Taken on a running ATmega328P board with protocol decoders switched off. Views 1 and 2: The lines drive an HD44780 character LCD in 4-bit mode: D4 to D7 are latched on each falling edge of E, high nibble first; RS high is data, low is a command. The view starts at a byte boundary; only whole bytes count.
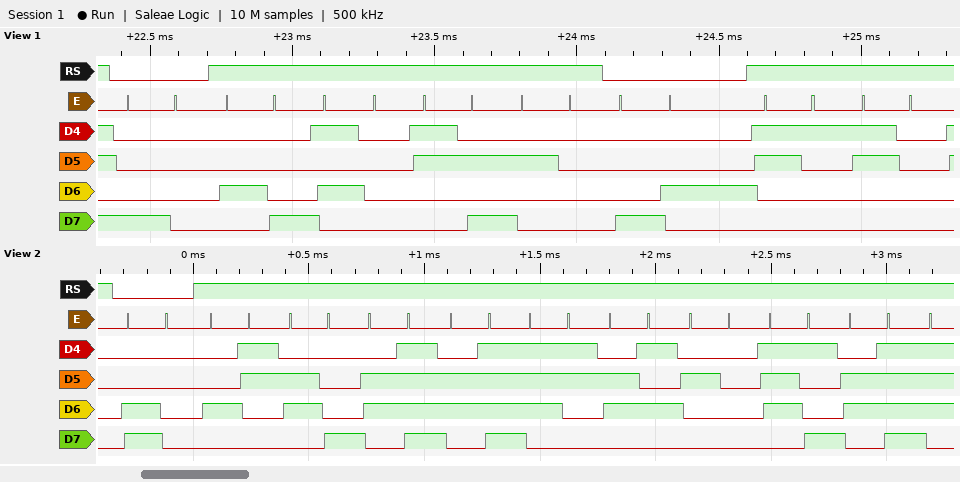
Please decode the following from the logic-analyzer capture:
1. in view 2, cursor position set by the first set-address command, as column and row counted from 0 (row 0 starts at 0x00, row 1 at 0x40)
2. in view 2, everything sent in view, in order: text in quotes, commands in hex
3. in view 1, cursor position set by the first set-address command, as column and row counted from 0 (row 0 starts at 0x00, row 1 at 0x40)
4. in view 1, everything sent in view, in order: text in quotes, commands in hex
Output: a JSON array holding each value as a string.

["column 0, row 1", "0xC0 \"Choose yo\"", "column 0, row 0", "0x80 \"HP: \" 0x84 \"10\""]
